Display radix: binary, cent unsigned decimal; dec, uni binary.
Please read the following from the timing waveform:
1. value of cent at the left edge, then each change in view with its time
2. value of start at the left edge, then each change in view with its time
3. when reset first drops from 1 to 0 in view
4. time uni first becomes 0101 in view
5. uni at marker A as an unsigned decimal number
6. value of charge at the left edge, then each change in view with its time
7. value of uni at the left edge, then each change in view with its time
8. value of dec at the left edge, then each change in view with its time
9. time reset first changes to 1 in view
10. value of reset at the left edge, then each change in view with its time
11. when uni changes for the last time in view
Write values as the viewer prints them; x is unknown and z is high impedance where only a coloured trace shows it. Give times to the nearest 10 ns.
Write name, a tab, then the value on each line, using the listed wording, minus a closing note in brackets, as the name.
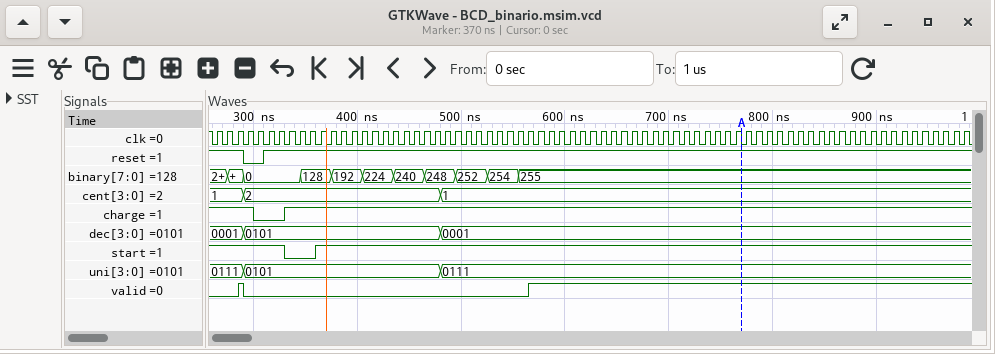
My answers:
value of cent at the left edge, then each change in view with its time	1, 2 at 290 ns, 1 at 480 ns
value of start at the left edge, then each change in view with its time	1, 0 at 330 ns, 1 at 360 ns
when reset first drops from 1 to 0 in view	290 ns
time uni first becomes 0101 in view	290 ns
uni at marker A as an unsigned decimal number	7
value of charge at the left edge, then each change in view with its time	1, 0 at 300 ns, 1 at 330 ns
value of uni at the left edge, then each change in view with its time	0111, 0101 at 290 ns, 0111 at 480 ns
value of dec at the left edge, then each change in view with its time	0001, 0101 at 290 ns, 0001 at 480 ns
time reset first changes to 1 in view	310 ns
value of reset at the left edge, then each change in view with its time	1, 0 at 290 ns, 1 at 310 ns
when uni changes for the last time in view	480 ns
